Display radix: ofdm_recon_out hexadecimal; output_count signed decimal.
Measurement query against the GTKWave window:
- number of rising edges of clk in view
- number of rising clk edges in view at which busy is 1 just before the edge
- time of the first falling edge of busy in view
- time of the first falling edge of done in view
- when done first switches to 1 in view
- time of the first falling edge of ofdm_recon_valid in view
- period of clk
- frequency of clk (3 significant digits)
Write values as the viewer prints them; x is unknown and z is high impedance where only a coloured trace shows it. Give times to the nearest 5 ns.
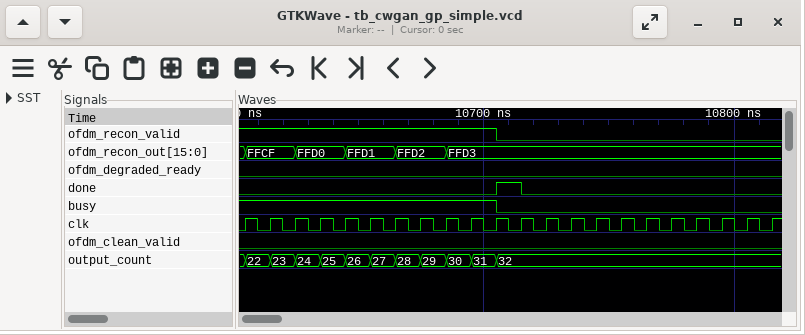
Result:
22
11
10705 ns
10715 ns
10705 ns
10705 ns
10 ns
100 MHz
